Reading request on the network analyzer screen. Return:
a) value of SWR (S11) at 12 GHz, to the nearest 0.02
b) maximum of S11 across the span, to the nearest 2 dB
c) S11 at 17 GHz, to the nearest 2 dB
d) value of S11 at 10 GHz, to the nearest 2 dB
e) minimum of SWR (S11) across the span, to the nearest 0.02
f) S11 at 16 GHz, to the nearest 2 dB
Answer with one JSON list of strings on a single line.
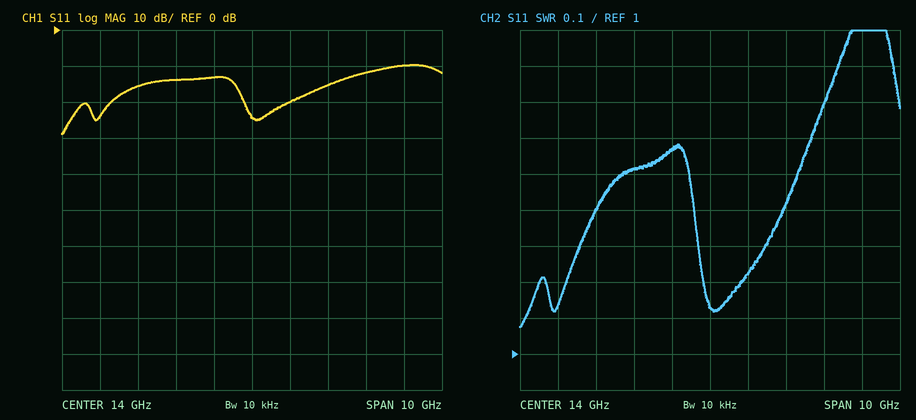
["1.52", "-10 dB", "-12 dB", "-24 dB", "1.08", "-16 dB"]
